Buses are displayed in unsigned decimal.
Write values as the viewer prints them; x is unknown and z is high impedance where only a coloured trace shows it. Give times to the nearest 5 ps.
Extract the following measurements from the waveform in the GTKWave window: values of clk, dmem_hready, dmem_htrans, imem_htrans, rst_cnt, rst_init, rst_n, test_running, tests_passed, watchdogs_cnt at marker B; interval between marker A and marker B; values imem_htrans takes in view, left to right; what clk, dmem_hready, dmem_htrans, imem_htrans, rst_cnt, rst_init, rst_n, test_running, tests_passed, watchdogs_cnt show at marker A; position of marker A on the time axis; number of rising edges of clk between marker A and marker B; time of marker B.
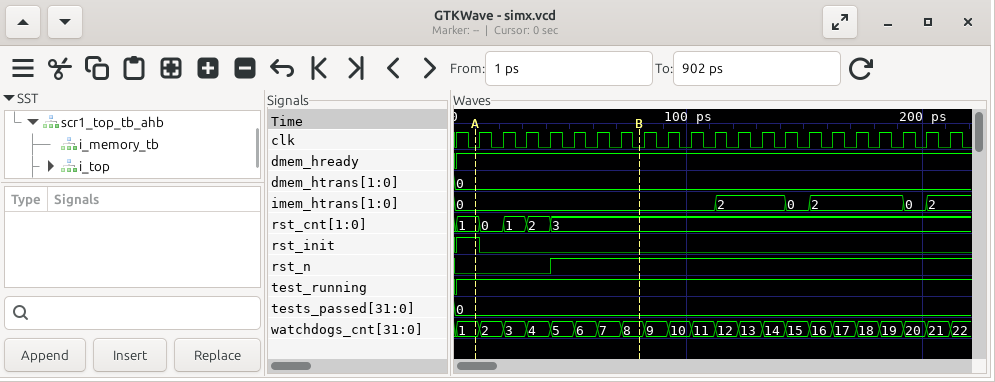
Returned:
clk=0, dmem_hready=1, dmem_htrans=0, imem_htrans=0, rst_cnt=3, rst_init=0, rst_n=1, test_running=1, tests_passed=0, watchdogs_cnt=8
70 ps
0, 2, 0, 2, 0, 2
clk=0, dmem_hready=1, dmem_htrans=0, imem_htrans=0, rst_cnt=1, rst_init=1, rst_n=0, test_running=1, tests_passed=0, watchdogs_cnt=1
10 ps
7
80 ps
